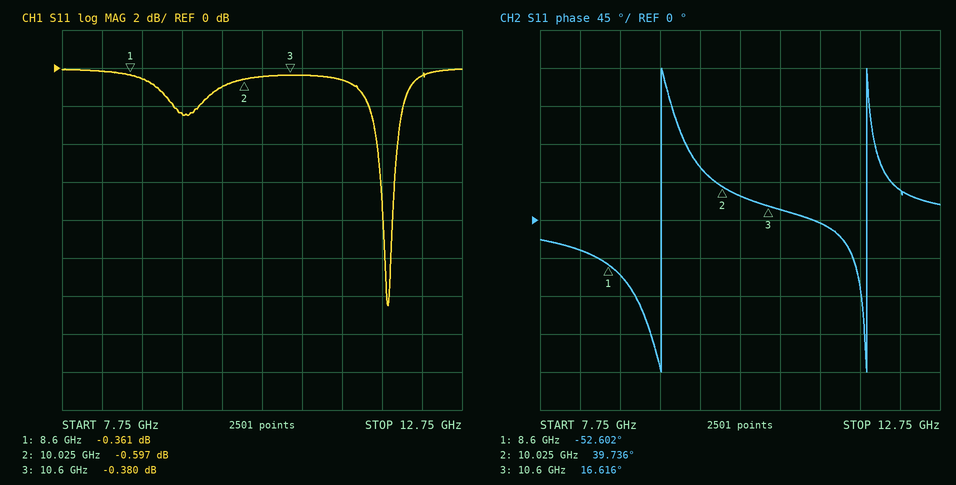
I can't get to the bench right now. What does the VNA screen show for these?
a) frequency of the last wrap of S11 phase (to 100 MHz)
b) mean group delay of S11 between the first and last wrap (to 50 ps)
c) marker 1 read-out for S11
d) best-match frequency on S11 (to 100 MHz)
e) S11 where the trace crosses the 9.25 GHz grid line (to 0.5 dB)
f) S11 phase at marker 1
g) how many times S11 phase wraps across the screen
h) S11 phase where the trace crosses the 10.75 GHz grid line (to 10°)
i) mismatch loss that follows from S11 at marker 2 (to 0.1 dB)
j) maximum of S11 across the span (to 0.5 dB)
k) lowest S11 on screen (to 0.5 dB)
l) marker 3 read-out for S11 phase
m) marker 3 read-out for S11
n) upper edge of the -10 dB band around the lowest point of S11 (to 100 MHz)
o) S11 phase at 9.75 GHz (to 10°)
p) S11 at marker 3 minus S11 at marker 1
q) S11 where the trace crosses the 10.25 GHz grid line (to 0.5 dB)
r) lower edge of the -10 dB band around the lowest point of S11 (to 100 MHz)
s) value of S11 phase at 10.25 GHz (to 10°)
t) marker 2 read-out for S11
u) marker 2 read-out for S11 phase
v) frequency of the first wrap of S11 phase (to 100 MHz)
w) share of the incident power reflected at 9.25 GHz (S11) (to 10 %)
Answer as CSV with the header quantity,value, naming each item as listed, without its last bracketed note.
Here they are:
quantity,value
frequency of the last wrap of S11 phase,11.8 GHz
mean group delay of S11 between the first and last wrap,400 ps
marker 1 read-out for S11,-0.361 dB
best-match frequency on S11,11.8 GHz
S11 where the trace crosses the 9.25 GHz grid line,-2.5 dB
S11 phase at marker 1,-52.602°
how many times S11 phase wraps across the screen,2
S11 phase where the trace crosses the 10.75 GHz grid line,10°
mismatch loss that follows from S11 at marker 2,8.9 dB
maximum of S11 across the span,0.0 dB
lowest S11 on screen,-12.5 dB
marker 3 read-out for S11 phase,16.616°
marker 3 read-out for S11,-0.380 dB
upper edge of the -10 dB band around the lowest point of S11,11.9 GHz
S11 phase at 9.75 GHz,60°
S11 at marker 3 minus S11 at marker 1,-0.019 dB
S11 where the trace crosses the 10.25 GHz grid line,-0.5 dB
lower edge of the -10 dB band around the lowest point of S11,11.8 GHz
value of S11 phase at 10.25 GHz,30°
marker 2 read-out for S11,-0.597 dB
marker 2 read-out for S11 phase,39.736°
frequency of the first wrap of S11 phase,9.3 GHz
share of the incident power reflected at 9.25 GHz (S11),60 %
